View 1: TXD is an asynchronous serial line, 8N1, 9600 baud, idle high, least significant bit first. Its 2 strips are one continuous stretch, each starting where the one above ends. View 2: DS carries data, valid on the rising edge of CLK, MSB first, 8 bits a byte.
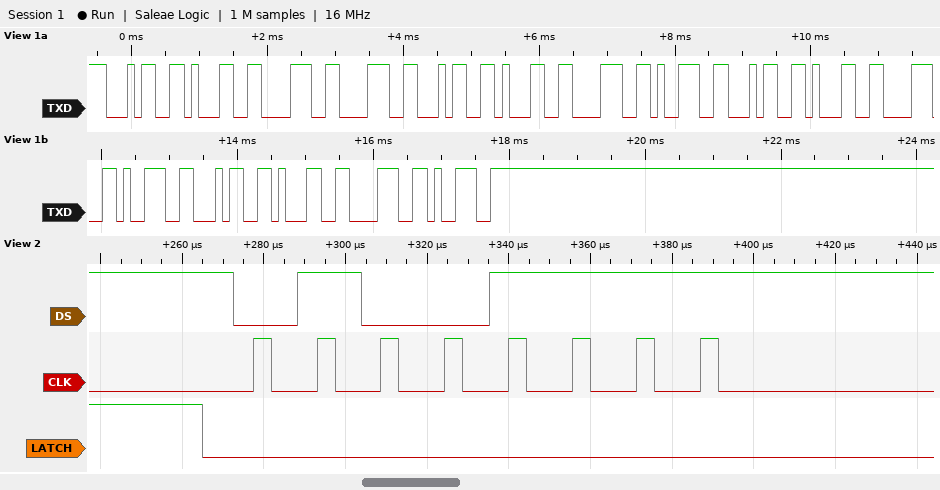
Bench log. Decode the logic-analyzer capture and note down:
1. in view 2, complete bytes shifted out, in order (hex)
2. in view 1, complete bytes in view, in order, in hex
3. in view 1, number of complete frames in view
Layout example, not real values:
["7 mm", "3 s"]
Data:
["4F", "34 31 38 38 34 31 38 39 34 31 38 39 34 31 38 39", "16"]
